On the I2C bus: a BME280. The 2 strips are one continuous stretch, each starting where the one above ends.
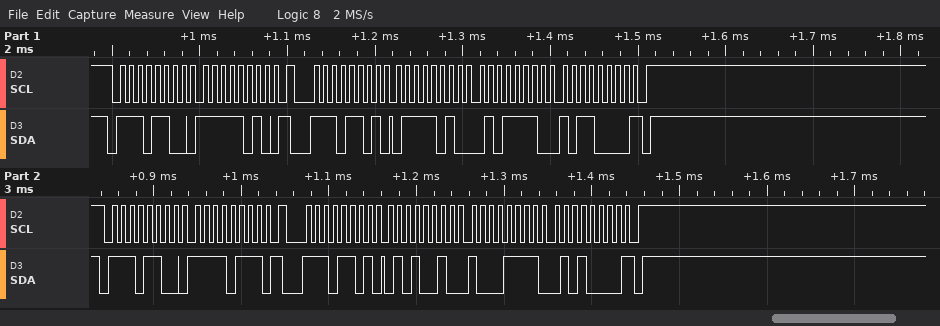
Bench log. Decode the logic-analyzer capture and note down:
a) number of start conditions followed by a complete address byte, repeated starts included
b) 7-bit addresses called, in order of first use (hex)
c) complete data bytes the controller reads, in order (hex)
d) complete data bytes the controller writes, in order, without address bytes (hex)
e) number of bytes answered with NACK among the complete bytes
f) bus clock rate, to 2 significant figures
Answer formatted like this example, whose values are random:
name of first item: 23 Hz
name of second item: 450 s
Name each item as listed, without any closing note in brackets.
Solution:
number of start conditions followed by a complete address byte, repeated starts included: 4
7-bit addresses called, in order of first use: 0x76
complete data bytes the controller reads, in order: 7A 5E B0 52 8F 50
complete data bytes the controller writes, in order, without address bytes: FA F7
number of bytes answered with NACK among the complete bytes: 2
bus clock rate, to 2 significant figures: 100 kHz
